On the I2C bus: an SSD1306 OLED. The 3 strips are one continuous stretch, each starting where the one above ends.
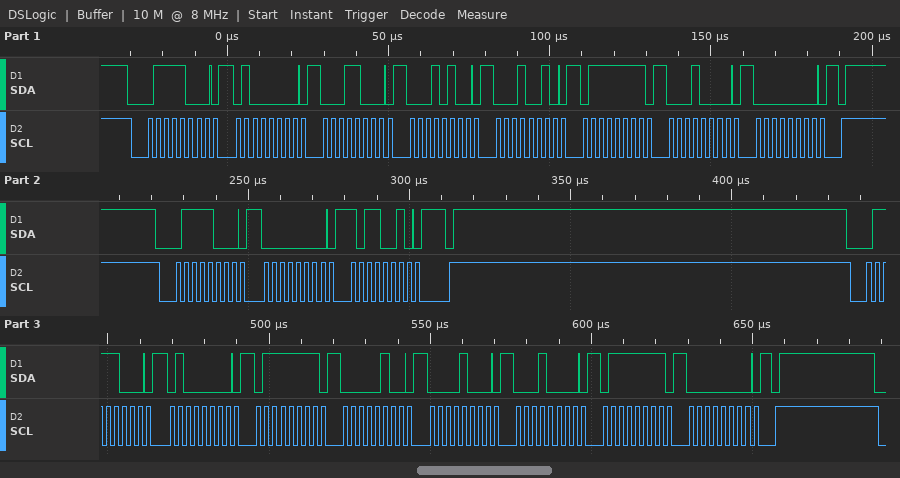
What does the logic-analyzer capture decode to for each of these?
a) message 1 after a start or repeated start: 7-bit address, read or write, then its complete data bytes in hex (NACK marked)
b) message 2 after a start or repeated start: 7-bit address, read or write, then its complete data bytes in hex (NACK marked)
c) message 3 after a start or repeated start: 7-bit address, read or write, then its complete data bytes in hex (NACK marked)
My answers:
0x3C write: 40 18 14 12 7F 10 00
0x3C write: 00 B2
0x3C write: 40 7F 04 08 10 7F 00
